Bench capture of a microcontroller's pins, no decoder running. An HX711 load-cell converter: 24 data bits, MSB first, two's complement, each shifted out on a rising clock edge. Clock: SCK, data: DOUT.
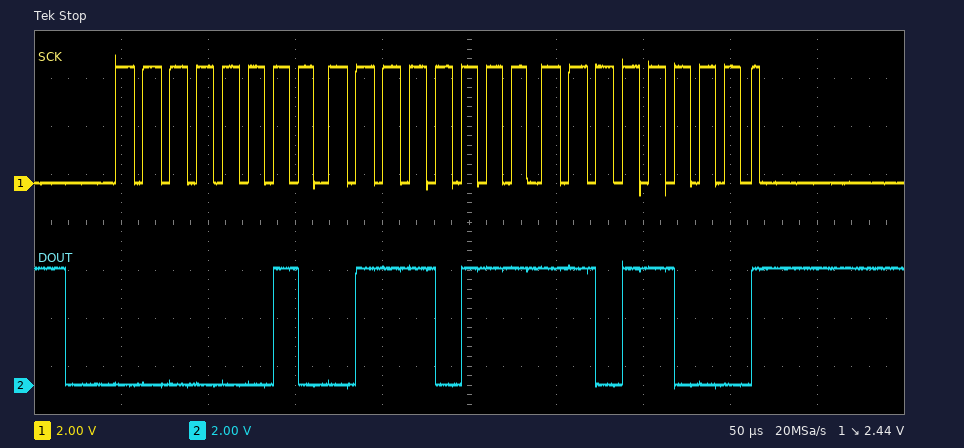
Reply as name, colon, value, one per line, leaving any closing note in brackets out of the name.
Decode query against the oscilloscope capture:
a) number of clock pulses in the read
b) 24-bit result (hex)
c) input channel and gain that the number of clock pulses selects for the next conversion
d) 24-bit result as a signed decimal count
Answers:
number of clock pulses in the read: 25
24-bit result: 0x0277D8
input channel and gain that the number of clock pulses selects for the next conversion: channel A, gain 128
24-bit result as a signed decimal count: 161752
